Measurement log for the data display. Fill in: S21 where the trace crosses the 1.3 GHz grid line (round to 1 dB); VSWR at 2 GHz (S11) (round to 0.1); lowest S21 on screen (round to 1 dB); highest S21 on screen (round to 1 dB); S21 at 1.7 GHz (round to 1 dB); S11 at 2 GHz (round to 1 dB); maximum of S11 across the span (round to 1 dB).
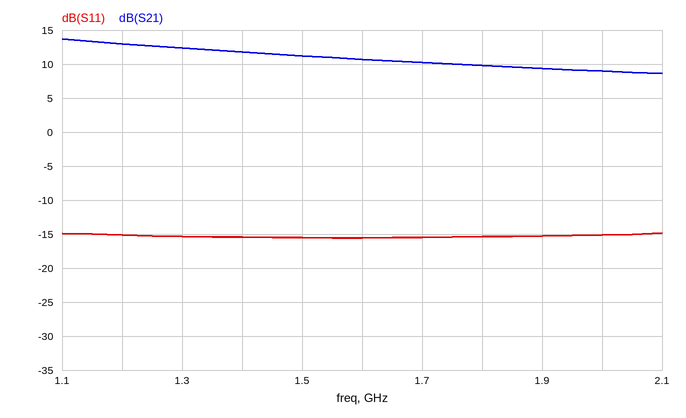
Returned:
12 dB
1.4
9 dB
14 dB
10 dB
-15 dB
-15 dB
